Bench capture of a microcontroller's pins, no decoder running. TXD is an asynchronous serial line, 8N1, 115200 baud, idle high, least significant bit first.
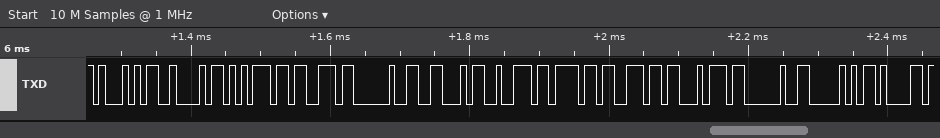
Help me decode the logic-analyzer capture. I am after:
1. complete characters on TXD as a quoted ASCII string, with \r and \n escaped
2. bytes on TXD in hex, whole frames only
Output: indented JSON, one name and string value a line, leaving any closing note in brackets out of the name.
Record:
{
  "complete characters on TXD as a quoted ASCII string, with \\r and \\n escaped": "\"QBus Front Pa\"",
  "bytes on TXD in hex, whole frames only": "0x51 0x42 0x75 0x73 0x20 0x46 0x72 0x6F 0x6E 0x74 0x20 0x50 0x61"
}
